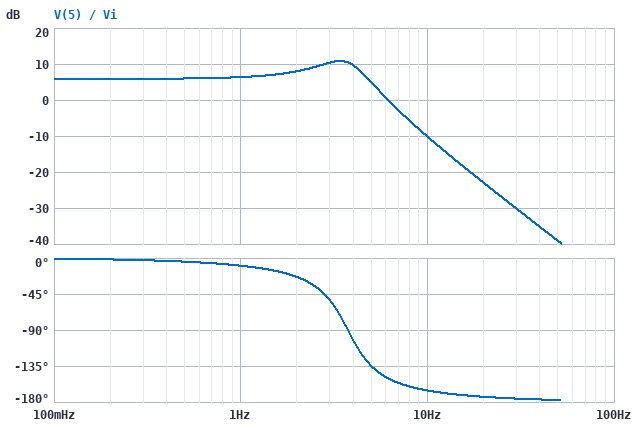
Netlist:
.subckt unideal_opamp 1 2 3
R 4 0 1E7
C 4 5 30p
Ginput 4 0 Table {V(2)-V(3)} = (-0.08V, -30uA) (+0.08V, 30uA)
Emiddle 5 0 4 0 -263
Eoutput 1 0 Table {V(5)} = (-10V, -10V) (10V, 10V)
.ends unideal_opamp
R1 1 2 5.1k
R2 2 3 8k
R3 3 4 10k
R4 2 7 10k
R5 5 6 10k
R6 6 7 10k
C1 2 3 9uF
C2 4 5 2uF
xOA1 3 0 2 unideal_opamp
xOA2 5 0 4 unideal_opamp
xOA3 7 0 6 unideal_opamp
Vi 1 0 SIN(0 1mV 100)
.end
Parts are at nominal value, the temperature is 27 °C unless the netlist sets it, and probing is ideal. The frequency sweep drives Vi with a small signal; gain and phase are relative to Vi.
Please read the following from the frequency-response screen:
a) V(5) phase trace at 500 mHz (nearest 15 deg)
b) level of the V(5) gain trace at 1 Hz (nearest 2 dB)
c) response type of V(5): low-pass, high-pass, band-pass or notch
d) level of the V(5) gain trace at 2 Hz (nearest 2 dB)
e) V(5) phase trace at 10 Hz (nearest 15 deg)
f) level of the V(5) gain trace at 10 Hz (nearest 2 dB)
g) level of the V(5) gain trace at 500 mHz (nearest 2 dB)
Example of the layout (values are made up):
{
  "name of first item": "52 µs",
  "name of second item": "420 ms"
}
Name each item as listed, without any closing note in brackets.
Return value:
{
  "V(5) phase trace at 500 mHz": "0 deg",
  "level of the V(5) gain trace at 1 Hz": "6 dB",
  "response type of V(5): low-pass, high-pass, band-pass or notch": "low-pass",
  "level of the V(5) gain trace at 2 Hz": "8 dB",
  "V(5) phase trace at 10 Hz": "-165 deg",
  "level of the V(5) gain trace at 10 Hz": "-10 dB",
  "level of the V(5) gain trace at 500 mHz": "6 dB"
}
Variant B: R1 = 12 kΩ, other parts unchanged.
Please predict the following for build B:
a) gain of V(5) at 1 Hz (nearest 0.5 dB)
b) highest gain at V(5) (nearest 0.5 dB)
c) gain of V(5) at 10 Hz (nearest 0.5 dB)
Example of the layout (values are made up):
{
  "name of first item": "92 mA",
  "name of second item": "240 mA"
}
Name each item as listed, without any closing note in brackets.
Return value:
{
  "gain of V(5) at 1 Hz": "-1.0 dB",
  "highest gain at V(5)": "3.5 dB",
  "gain of V(5) at 10 Hz": "-17.5 dB"
}
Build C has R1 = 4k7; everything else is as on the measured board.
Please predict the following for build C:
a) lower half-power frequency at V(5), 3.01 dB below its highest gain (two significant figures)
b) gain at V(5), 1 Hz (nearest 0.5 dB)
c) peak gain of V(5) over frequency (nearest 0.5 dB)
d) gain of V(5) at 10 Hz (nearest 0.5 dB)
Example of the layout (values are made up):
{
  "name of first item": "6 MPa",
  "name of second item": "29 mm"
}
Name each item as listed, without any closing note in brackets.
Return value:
{
  "lower half-power frequency at V(5), 3.01 dB below its highest gain": "1.9 Hz",
  "gain at V(5), 1 Hz": "7.0 dB",
  "peak gain of V(5) over frequency": "11.5 dB",
  "gain of V(5) at 10 Hz": "-9.5 dB"
}
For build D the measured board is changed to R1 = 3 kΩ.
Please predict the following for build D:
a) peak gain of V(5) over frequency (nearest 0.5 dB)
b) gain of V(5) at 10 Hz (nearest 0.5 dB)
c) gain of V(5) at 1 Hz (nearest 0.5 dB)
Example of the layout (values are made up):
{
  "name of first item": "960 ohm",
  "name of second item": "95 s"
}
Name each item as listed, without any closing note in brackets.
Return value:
{
  "peak gain of V(5) over frequency": "15.5 dB",
  "gain of V(5) at 10 Hz": "-5.5 dB",
  "gain of V(5) at 1 Hz": "11.0 dB"
}
